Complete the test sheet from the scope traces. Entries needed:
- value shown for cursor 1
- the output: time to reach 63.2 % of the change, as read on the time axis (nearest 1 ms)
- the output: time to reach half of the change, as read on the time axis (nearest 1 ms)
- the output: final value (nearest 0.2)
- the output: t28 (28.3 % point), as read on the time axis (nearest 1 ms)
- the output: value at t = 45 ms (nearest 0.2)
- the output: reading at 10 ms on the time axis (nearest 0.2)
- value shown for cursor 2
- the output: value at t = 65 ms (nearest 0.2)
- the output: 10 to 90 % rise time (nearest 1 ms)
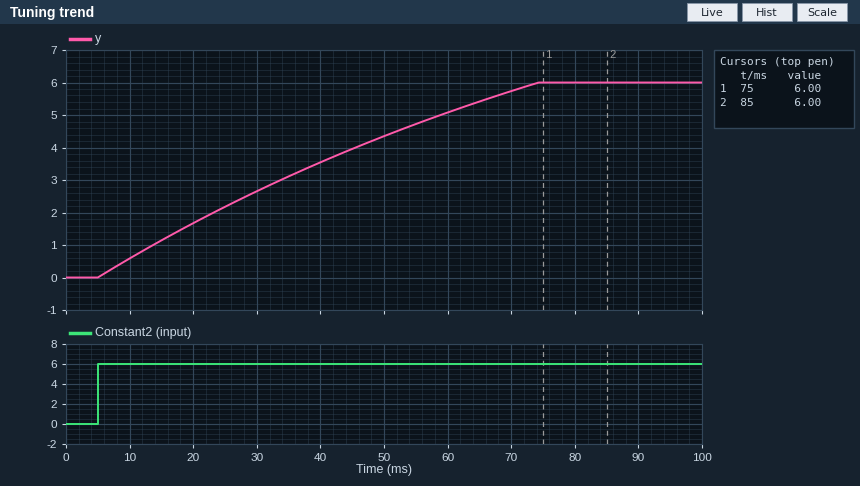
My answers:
6.00
43 ms
34 ms
6.0
20 ms
4.0
0.6
6.00
5.4
55 ms
